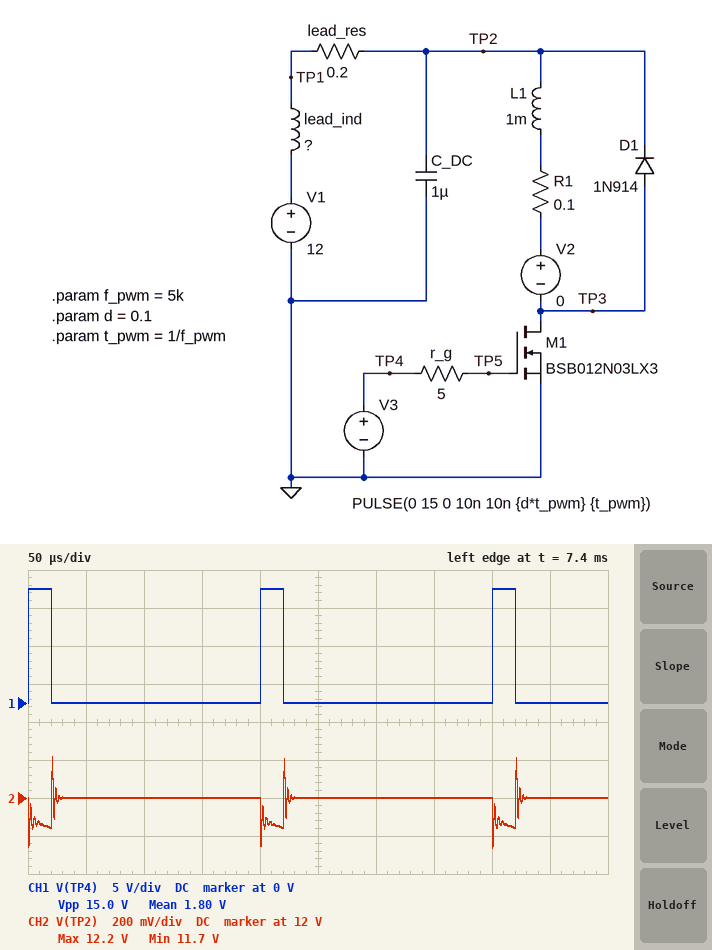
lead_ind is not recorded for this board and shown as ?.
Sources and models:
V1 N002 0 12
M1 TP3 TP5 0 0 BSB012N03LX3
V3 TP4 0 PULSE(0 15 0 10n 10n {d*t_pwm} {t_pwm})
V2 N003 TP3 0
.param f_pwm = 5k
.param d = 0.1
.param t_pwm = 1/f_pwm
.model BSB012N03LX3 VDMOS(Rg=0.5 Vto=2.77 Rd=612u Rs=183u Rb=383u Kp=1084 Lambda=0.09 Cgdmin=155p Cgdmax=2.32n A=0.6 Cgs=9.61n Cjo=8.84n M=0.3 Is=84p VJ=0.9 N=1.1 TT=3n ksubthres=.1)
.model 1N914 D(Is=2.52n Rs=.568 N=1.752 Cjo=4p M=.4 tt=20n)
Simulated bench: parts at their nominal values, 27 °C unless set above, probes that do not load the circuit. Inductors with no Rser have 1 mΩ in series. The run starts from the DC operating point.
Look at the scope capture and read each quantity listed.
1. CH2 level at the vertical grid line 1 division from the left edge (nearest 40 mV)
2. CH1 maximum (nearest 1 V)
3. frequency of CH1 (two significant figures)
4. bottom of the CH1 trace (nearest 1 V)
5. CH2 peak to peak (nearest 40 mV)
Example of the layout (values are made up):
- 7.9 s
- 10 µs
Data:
- 12.00 V
- 15 V
- 5.0 kHz
- 0 V
- 480 mV
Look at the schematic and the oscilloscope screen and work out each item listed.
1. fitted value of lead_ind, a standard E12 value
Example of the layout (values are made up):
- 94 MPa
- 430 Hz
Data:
- 180 nH
